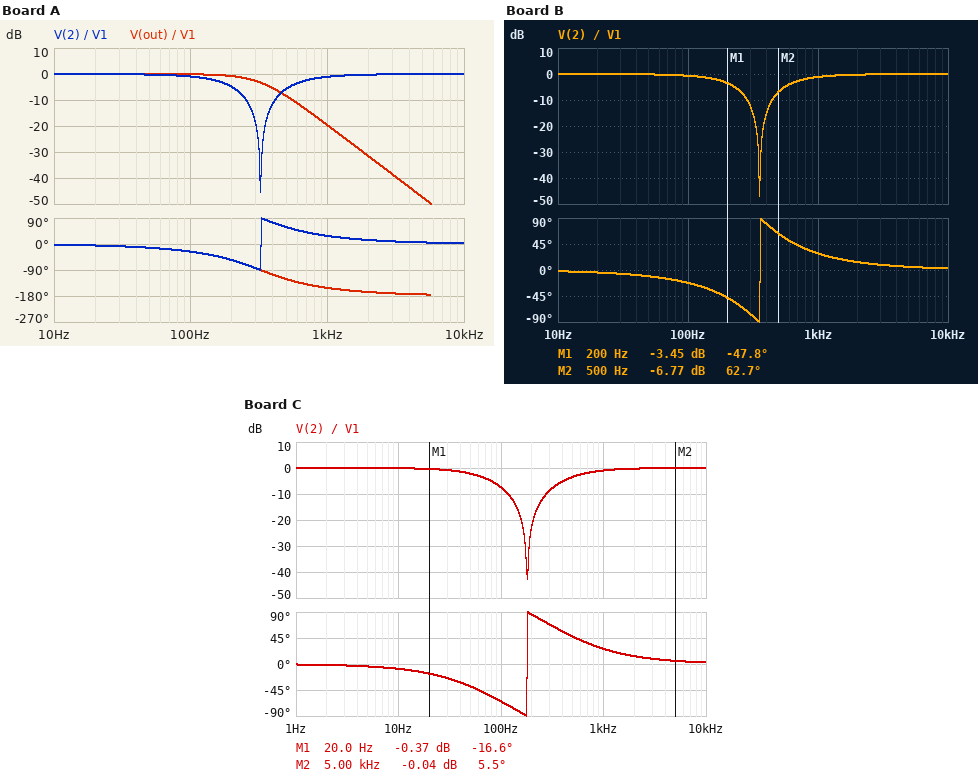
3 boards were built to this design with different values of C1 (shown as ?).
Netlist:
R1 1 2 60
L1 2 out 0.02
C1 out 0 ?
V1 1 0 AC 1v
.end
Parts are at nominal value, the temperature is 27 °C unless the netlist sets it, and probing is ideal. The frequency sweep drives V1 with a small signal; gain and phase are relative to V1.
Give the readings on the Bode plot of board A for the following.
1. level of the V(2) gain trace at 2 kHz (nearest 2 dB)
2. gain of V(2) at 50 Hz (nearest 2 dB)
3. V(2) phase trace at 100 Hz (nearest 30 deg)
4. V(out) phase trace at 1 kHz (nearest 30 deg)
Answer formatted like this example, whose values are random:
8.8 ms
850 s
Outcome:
0 dB
0 dB
-30 deg
-150 deg
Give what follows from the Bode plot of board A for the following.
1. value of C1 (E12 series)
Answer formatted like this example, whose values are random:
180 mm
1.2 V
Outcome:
12 µF
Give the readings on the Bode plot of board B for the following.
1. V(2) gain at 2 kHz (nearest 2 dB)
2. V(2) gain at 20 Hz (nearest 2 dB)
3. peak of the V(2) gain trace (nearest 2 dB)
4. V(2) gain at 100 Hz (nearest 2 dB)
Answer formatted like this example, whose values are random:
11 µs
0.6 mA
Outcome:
0 dB
0 dB
0 dB
0 dB
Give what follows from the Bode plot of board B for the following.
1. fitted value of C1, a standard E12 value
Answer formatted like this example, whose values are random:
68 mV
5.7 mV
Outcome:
10 µF
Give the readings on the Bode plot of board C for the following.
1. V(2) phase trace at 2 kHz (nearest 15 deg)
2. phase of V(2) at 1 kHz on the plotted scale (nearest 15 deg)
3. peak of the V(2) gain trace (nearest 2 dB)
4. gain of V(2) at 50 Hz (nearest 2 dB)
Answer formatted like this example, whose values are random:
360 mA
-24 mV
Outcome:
15 deg
30 deg
0 dB
-2 dB
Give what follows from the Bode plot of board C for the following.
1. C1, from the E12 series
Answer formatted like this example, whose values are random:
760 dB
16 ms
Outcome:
39 µF
